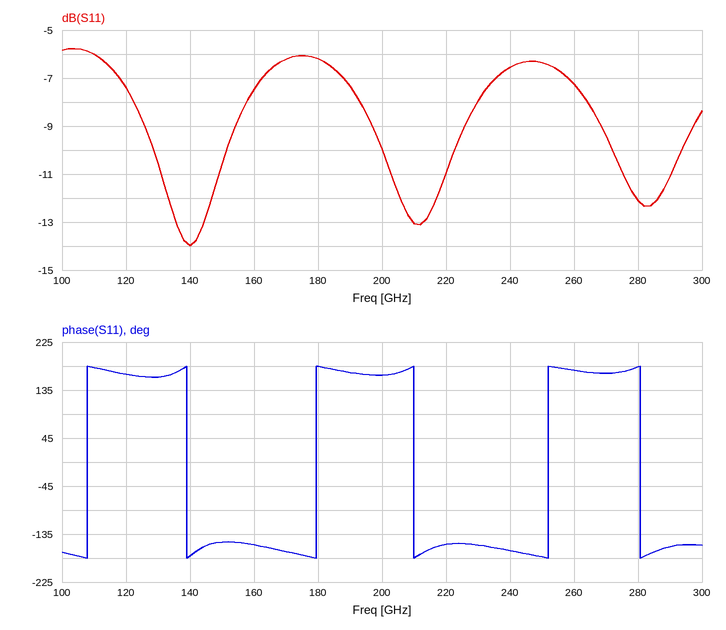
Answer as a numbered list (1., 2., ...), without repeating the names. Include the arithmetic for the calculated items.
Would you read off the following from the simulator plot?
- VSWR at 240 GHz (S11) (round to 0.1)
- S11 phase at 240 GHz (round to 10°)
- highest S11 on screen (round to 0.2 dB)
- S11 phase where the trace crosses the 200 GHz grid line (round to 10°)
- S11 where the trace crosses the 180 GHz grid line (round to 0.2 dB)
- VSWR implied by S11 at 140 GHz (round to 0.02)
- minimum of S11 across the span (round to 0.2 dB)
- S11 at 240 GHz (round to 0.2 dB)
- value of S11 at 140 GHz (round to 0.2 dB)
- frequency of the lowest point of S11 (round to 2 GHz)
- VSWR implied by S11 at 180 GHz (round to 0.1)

1. |Γ| = 10^(-6.6/20) = 0.4677; VSWR = (1 + 0.4677)/(1 − 0.4677) ≈ 2.8
2. -170°
3. -5.8 dB
4. 160°
5. -6.2 dB
6. |Γ| = 10^(-14/20) = 0.1995; VSWR = (1 + 0.1995)/(1 − 0.1995) ≈ 1.50
7. -14.0 dB
8. -6.6 dB
9. -14.0 dB
10. 140 GHz
11. |Γ| = 10^(-6.2/20) = 0.4898; VSWR = (1 + 0.4898)/(1 − 0.4898) ≈ 2.9
